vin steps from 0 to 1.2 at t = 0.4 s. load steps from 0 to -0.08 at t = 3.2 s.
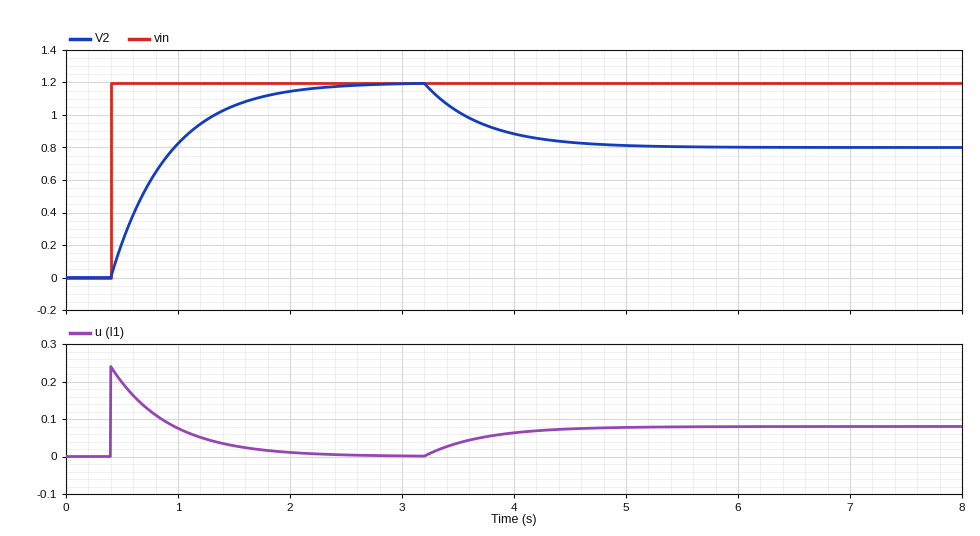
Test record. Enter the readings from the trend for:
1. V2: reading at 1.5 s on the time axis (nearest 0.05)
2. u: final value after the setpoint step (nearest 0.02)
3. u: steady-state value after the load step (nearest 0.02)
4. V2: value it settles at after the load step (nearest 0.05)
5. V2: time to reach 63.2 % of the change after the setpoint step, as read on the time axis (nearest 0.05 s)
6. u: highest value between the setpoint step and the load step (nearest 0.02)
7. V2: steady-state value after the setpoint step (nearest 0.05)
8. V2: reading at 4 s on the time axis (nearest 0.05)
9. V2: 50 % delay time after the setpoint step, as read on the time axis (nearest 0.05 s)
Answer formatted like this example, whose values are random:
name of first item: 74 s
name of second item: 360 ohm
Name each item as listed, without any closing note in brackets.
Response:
V2: reading at 1.5 s on the time axis: 1.05
u: final value after the setpoint step: 0.00
u: steady-state value after the load step: 0.08
V2: value it settles at after the load step: 0.80
V2: time to reach 63.2 % of the change after the setpoint step, as read on the time axis: 0.90 s
u: highest value between the setpoint step and the load step: 0.24
V2: steady-state value after the setpoint step: 1.20
V2: reading at 4 s on the time axis: 0.90
V2: 50 % delay time after the setpoint step, as read on the time axis: 0.75 s
